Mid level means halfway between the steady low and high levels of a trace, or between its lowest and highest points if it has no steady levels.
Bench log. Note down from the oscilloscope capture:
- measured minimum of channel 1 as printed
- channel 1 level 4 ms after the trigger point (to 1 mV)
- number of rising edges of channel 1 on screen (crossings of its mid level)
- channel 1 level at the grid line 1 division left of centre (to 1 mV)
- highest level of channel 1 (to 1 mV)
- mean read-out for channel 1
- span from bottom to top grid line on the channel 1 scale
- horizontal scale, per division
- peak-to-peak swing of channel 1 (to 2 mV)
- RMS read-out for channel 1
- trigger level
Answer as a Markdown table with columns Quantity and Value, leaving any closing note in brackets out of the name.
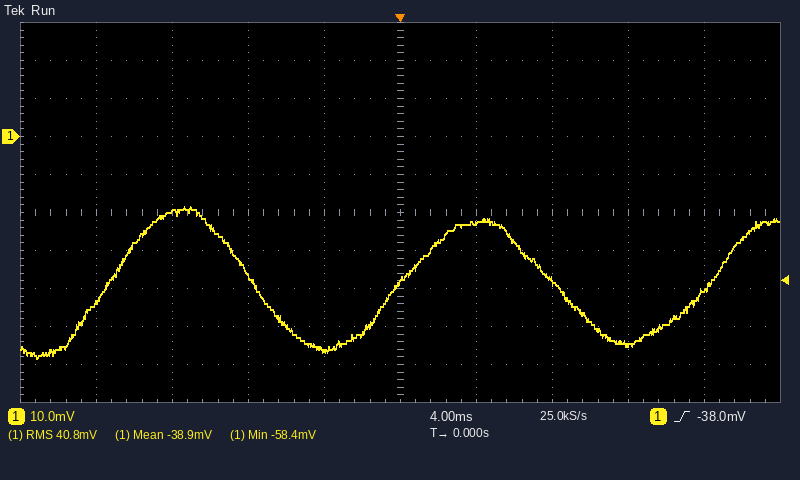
| Quantity | Value |
|---|---|
| measured minimum of channel 1 as printed | -58.4 mV |
| channel 1 level 4 ms after the trigger point | -23 mV |
| number of rising edges of channel 1 on screen | 3 |
| channel 1 level at the grid line 1 division left of centre | -56 mV |
| highest level of channel 1 | -18 mV |
| mean read-out for channel 1 | -38.9 mV |
| span from bottom to top grid line on the channel 1 scale | 100 mV |
| horizontal scale, per division | 4 ms |
| peak-to-peak swing of channel 1 | 40 mV |
| RMS read-out for channel 1 | 40.8 mV |
| trigger level | -38.0 mV |
